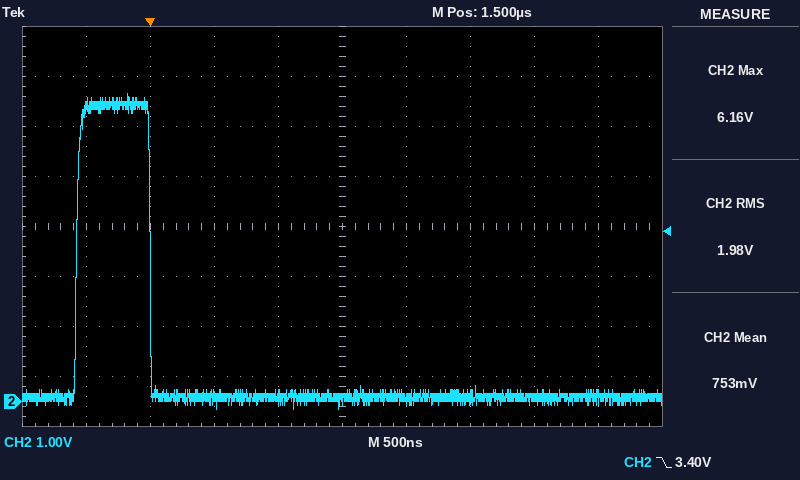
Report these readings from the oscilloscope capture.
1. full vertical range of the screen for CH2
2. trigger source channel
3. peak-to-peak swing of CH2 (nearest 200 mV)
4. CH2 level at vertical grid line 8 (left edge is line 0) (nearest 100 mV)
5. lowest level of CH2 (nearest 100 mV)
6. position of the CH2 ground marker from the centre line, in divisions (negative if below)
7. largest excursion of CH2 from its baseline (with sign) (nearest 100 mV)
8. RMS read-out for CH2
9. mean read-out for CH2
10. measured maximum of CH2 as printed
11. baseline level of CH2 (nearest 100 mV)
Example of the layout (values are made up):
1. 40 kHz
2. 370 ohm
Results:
1. 8 V
2. CH2
3. 6.4 V
4. 100 mV
5. -200 mV
6. -3.5 div
7. +6.1 V
8. 1.98 V
9. 753 mV
10. 6.16 V
11. 100 mV
